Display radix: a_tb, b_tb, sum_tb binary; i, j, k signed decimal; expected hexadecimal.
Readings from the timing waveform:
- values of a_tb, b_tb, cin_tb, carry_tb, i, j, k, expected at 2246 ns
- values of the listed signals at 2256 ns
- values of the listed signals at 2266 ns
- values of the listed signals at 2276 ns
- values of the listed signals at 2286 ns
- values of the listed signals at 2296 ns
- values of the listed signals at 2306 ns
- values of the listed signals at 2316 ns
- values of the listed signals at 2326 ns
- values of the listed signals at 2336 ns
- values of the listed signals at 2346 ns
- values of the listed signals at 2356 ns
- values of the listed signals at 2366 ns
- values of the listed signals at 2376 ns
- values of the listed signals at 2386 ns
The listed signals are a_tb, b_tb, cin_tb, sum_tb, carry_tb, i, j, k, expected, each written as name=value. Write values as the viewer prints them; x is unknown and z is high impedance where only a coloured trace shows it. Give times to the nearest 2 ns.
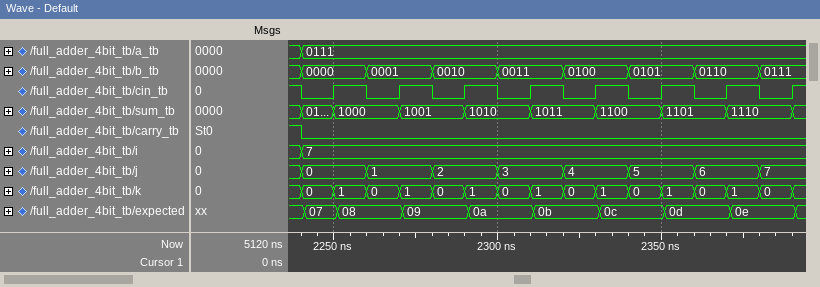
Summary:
a_tb=0111, b_tb=0000, cin_tb=0, carry_tb=0, i=7, j=0, k=0, expected=07
a_tb=0111, b_tb=0000, cin_tb=1, sum_tb=1000, carry_tb=0, i=7, j=0, k=1, expected=08
a_tb=0111, b_tb=0001, cin_tb=0, sum_tb=1000, carry_tb=0, i=7, j=1, k=0, expected=08
a_tb=0111, b_tb=0001, cin_tb=1, sum_tb=1001, carry_tb=0, i=7, j=1, k=1, expected=09
a_tb=0111, b_tb=0010, cin_tb=0, sum_tb=1001, carry_tb=0, i=7, j=2, k=0, expected=09
a_tb=0111, b_tb=0010, cin_tb=1, sum_tb=1010, carry_tb=0, i=7, j=2, k=1, expected=0a
a_tb=0111, b_tb=0011, cin_tb=0, sum_tb=1010, carry_tb=0, i=7, j=3, k=0, expected=0a
a_tb=0111, b_tb=0011, cin_tb=1, sum_tb=1011, carry_tb=0, i=7, j=3, k=1, expected=0b
a_tb=0111, b_tb=0100, cin_tb=0, sum_tb=1011, carry_tb=0, i=7, j=4, k=0, expected=0b
a_tb=0111, b_tb=0100, cin_tb=1, sum_tb=1100, carry_tb=0, i=7, j=4, k=1, expected=0c
a_tb=0111, b_tb=0101, cin_tb=0, sum_tb=1100, carry_tb=0, i=7, j=5, k=0, expected=0c
a_tb=0111, b_tb=0101, cin_tb=1, sum_tb=1101, carry_tb=0, i=7, j=5, k=1, expected=0d
a_tb=0111, b_tb=0110, cin_tb=0, sum_tb=1101, carry_tb=0, i=7, j=6, k=0, expected=0d
a_tb=0111, b_tb=0110, cin_tb=1, sum_tb=1110, carry_tb=0, i=7, j=6, k=1, expected=0e
a_tb=0111, b_tb=0111, cin_tb=0, sum_tb=1110, carry_tb=0, i=7, j=7, k=0, expected=0e
